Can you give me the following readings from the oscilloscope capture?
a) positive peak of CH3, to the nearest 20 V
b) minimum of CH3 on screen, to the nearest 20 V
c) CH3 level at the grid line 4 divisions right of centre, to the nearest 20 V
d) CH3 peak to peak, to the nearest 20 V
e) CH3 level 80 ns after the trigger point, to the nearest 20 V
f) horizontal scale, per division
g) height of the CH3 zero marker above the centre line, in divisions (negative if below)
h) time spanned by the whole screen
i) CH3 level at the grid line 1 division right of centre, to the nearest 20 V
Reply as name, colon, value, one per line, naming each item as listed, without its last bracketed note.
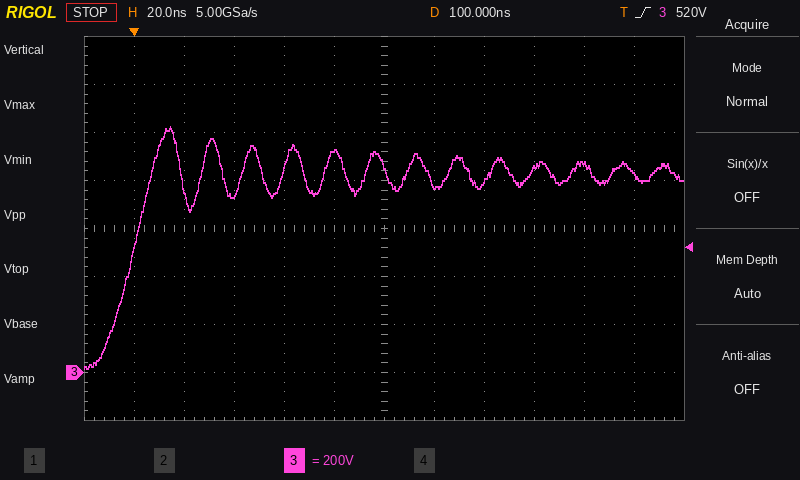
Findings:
positive peak of CH3, to the nearest 20 V: 1.02 kV
minimum of CH3 on screen, to the nearest 20 V: 20 V
CH3 level at the grid line 4 divisions right of centre, to the nearest 20 V: 860 V
CH3 peak to peak, to the nearest 20 V: 1.00 kV
CH3 level 80 ns after the trigger point, to the nearest 20 V: 920 V
horizontal scale, per division: 20 ns
height of the CH3 zero marker above the centre line, in divisions: -3.0 div
time spanned by the whole screen: 240 ns
CH3 level at the grid line 1 division right of centre, to the nearest 20 V: 780 V
